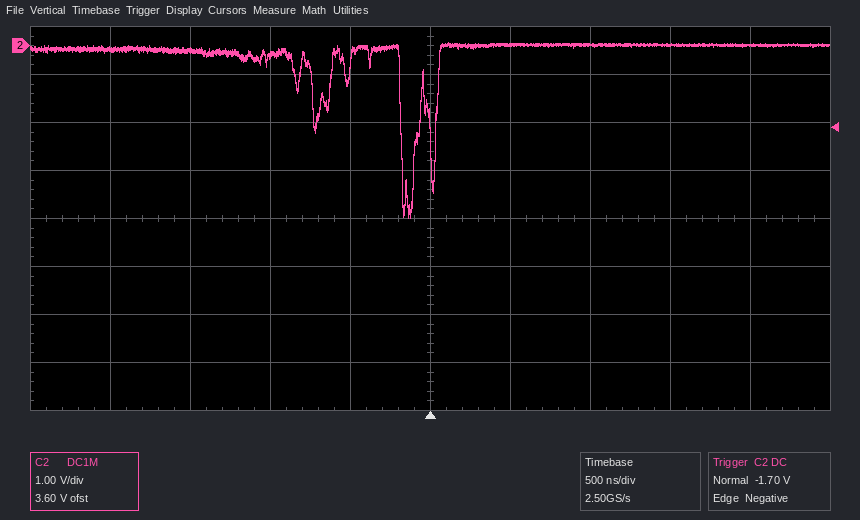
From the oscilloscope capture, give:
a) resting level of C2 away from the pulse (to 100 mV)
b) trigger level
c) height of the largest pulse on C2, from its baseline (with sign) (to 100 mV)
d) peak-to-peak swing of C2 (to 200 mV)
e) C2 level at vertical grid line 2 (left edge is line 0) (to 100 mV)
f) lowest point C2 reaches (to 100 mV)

0.0 V
-1.70 V
-3.6 V
3.6 V
-100 mV
-3.6 V
